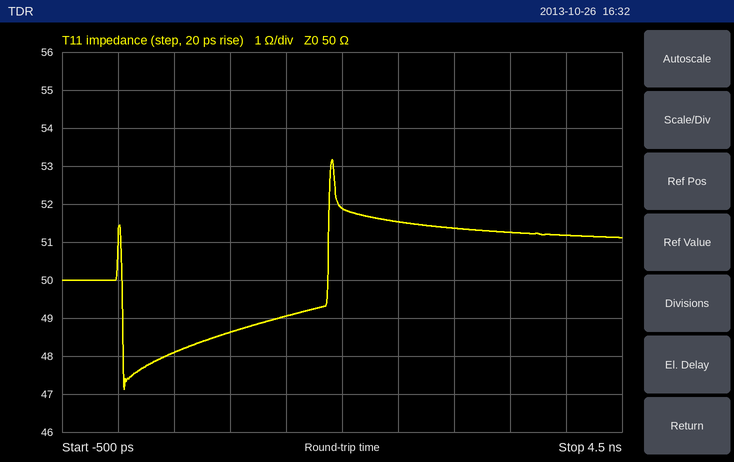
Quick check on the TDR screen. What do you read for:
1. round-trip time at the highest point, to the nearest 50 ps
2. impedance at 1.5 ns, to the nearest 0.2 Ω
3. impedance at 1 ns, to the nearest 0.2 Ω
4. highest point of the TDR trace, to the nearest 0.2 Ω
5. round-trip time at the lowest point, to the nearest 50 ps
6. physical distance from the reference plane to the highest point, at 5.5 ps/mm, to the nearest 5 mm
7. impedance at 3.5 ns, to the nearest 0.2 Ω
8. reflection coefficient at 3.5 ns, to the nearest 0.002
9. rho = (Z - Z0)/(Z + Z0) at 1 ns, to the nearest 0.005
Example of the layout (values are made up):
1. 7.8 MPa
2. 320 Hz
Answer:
1. 1.90 ns
2. 49.0 Ω
3. 48.6 Ω
4. 53.2 Ω
5. 50 ps
6. 175 mm
7. 51.2 Ω
8. +0.012
9. -0.015
